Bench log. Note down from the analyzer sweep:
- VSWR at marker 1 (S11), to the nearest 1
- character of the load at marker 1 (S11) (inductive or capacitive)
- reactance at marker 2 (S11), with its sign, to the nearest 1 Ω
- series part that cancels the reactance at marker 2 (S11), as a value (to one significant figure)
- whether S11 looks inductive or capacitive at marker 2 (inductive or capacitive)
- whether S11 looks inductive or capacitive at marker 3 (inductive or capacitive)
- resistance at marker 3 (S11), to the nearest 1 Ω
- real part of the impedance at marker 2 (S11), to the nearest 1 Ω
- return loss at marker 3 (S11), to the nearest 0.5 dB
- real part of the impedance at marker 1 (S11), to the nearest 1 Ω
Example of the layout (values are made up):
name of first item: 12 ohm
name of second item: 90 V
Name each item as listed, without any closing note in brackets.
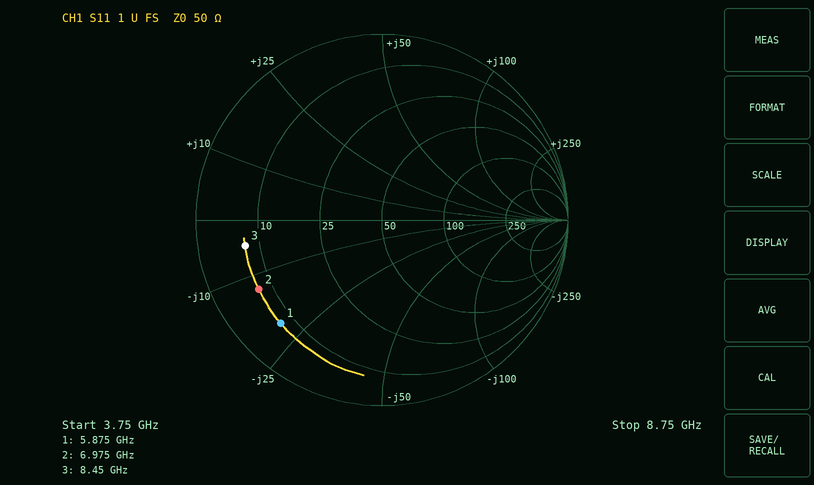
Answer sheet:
VSWR at marker 1 (S11), to the nearest 1: 8
character of the load at marker 1 (S11): capacitive
reactance at marker 2 (S11), with its sign, to the nearest 1 Ω: -13 Ω
series part that cancels the reactance at marker 2 (S11), as a value: 300 pH
whether S11 looks inductive or capacitive at marker 2: capacitive
whether S11 looks inductive or capacitive at marker 3: capacitive
resistance at marker 3 (S11), to the nearest 1 Ω: 7 Ω
real part of the impedance at marker 2 (S11), to the nearest 1 Ω: 7 Ω
return loss at marker 3 (S11), to the nearest 0.5 dB: 2.5 dB
real part of the impedance at marker 1 (S11), to the nearest 1 Ω: 7 Ω
